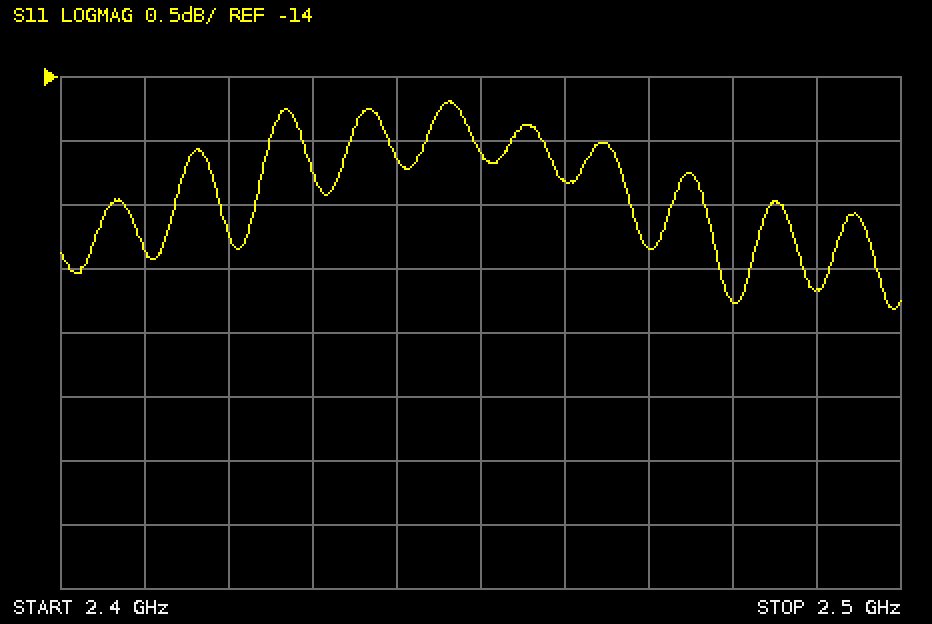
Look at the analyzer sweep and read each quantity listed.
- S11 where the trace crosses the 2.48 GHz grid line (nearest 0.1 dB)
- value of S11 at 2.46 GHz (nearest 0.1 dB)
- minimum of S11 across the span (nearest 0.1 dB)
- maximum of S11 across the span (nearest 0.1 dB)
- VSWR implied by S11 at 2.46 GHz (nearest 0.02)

-15.8 dB
-14.8 dB
-15.8 dB
-14.2 dB
1.44
